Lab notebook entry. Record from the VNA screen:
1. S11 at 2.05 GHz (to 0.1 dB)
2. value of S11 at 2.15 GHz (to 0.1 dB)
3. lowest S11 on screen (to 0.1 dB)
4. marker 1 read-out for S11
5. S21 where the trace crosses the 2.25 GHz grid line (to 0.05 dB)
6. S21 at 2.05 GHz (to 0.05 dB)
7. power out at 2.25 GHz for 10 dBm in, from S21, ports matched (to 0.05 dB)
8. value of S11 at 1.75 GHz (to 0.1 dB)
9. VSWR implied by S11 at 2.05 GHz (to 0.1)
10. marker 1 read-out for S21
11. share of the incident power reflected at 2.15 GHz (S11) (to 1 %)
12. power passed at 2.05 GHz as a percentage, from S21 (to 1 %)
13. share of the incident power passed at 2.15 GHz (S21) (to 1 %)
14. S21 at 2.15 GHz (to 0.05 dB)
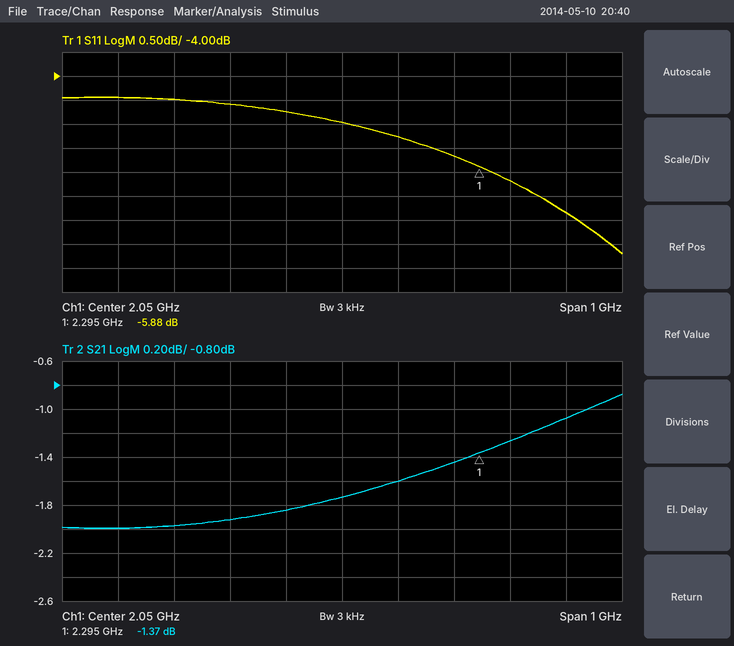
-5.0 dB
-5.3 dB
-7.7 dB
-5.88 dB
-1.45 dB
-1.75 dB
8.55 dBm
-4.5 dB
3.6
-1.37 dB
30 %
67 %
69 %
-1.60 dB
